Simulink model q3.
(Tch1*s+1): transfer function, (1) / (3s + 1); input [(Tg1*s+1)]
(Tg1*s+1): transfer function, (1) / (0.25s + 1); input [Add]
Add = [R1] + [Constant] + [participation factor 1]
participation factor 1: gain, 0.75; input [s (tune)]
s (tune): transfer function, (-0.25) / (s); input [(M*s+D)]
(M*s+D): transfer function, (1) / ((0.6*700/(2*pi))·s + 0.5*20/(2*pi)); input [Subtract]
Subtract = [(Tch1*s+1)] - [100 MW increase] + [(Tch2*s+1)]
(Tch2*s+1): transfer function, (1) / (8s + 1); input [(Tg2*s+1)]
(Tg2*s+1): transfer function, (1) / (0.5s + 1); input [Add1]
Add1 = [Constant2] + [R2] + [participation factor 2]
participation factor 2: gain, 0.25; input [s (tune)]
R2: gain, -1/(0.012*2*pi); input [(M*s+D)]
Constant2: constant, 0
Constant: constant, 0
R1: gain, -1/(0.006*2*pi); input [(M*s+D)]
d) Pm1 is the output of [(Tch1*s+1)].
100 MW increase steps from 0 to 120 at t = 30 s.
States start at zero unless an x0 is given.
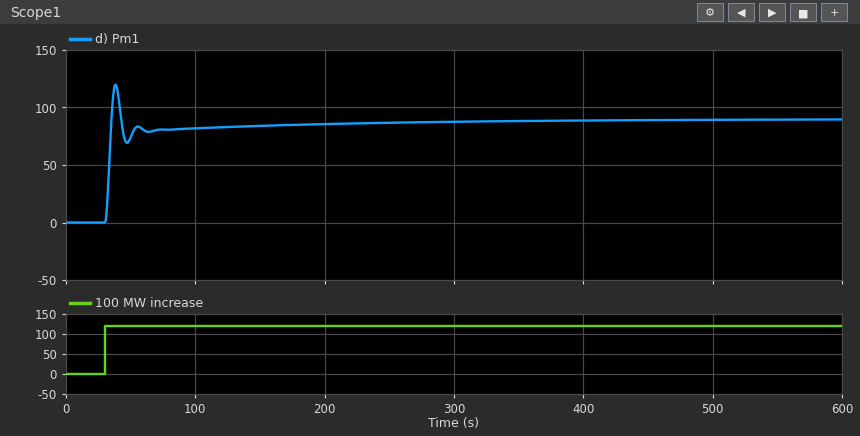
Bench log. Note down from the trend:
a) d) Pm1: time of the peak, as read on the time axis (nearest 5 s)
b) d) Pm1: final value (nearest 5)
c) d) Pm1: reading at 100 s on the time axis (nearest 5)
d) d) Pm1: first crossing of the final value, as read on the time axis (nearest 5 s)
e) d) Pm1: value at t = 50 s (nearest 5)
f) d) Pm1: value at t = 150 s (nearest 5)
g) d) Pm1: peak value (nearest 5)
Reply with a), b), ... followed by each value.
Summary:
a) 40 s
b) 90
c) 80
d) 35 s
e) 75
f) 85
g) 120
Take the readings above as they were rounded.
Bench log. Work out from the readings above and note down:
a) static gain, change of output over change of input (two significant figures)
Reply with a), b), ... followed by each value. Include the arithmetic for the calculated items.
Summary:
a) (90 - 0) / (120 - 0) = 0.75
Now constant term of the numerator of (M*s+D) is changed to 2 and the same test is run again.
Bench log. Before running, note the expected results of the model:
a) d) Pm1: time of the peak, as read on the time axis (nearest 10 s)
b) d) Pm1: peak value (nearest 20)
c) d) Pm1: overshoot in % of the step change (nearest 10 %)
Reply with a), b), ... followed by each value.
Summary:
a) 40 s
b) 140
c) 60 %
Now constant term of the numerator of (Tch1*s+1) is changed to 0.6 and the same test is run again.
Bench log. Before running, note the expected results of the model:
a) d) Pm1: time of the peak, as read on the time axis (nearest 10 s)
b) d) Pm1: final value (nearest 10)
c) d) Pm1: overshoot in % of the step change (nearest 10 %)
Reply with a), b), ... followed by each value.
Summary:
a) 40 s
b) 80
c) 20 %
